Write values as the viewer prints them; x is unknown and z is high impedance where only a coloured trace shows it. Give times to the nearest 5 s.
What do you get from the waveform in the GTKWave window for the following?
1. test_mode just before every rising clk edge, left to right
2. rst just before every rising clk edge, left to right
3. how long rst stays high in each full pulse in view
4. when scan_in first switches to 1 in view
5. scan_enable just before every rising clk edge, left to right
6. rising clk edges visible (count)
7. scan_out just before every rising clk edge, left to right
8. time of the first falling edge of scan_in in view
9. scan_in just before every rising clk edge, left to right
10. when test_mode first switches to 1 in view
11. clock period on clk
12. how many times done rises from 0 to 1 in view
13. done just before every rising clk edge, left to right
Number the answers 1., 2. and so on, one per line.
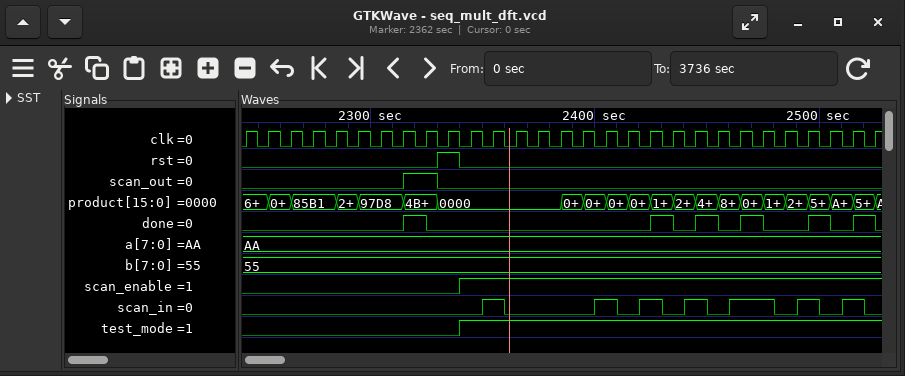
1. 0 0 0 0 0 0 0 0 0 0 1 1 1 1 1 1 1 1 1 1 1 1 1 1 1 1 1 1 1
2. 0 0 0 0 0 0 0 0 0 1 0 0 0 0 0 0 0 0 0 0 0 0 0 0 0 0 0 0 0
3. 10 s
4. 2350 s
5. 0 0 0 0 0 0 0 0 0 0 1 1 1 1 1 1 1 1 1 1 1 1 1 1 1 1 1 1 1
6. 29
7. 0 0 0 0 0 0 0 0 1 0 0 0 0 0 0 0 0 0 0 0 0 0 0 0 0 0 0 0 0
8. 2360 s
9. 0 0 0 0 0 0 0 0 0 0 0 1 0 0 0 0 1 0 1 0 1 0 1 1 0 1 0 1 0
10. 2340 s
11. 10 s
12. 6
13. 0 0 0 0 0 0 0 0 1 0 0 0 0 0 0 0 0 0 0 1 0 1 0 1 0 0 1 0 1
